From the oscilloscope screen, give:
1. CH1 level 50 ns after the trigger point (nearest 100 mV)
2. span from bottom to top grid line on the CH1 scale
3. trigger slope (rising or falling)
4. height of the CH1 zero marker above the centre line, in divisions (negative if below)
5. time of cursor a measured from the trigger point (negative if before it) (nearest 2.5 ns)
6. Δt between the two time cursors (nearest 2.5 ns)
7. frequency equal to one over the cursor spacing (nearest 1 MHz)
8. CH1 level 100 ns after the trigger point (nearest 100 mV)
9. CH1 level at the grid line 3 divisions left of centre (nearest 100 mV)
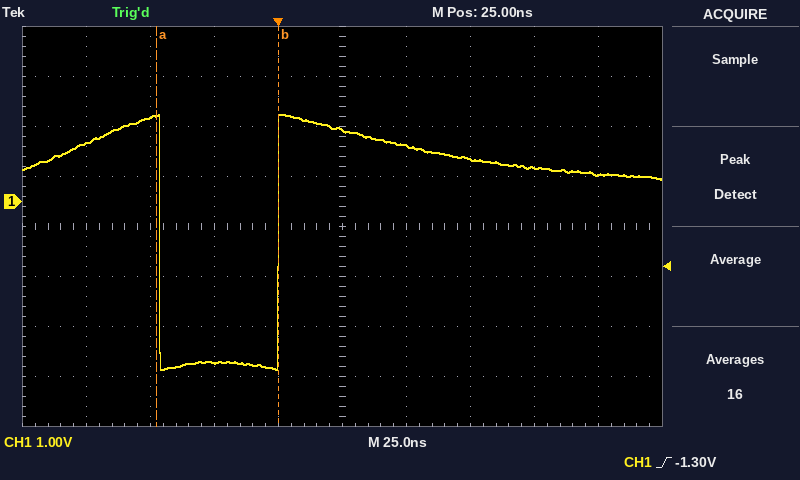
1.1 V
8 V
rising
+0.5 div
-47.5 ns
47.5 ns
21 MHz
700 mV
1.7 V
